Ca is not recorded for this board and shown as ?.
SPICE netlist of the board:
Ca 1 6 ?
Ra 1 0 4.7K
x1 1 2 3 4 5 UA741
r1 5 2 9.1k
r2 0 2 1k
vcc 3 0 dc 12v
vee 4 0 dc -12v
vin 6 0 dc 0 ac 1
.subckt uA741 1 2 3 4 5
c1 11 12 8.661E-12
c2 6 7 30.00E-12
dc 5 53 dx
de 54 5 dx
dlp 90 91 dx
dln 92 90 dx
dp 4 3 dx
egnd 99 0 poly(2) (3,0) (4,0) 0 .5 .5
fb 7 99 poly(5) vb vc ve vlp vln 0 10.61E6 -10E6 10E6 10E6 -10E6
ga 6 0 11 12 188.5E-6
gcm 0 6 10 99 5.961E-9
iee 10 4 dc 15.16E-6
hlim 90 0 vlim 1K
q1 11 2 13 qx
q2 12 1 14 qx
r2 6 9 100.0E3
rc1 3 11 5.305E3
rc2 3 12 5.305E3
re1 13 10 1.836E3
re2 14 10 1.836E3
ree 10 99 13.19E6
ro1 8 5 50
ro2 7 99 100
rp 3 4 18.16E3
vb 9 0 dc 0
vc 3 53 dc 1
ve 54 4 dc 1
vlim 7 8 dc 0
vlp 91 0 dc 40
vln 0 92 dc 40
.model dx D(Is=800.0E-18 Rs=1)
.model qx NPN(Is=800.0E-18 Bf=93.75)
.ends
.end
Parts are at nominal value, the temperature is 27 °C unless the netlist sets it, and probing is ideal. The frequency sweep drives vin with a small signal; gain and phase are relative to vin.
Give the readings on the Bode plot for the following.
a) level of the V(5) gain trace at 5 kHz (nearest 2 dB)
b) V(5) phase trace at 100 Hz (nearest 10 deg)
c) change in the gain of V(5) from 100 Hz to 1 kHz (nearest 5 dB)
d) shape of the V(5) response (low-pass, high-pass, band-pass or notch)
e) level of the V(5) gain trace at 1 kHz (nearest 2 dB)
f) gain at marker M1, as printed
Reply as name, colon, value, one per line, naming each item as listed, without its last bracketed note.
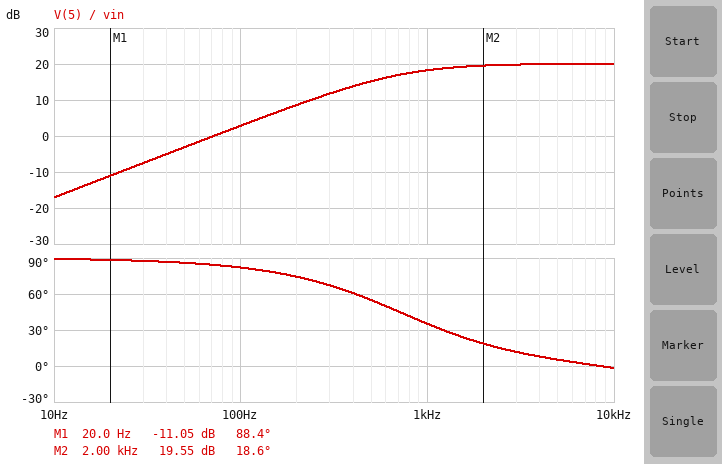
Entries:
level of the V(5) gain trace at 5 kHz: 20 dB
V(5) phase trace at 100 Hz: 80 deg
change in the gain of V(5) from 100 Hz to 1 kHz: 15 dB
shape of the V(5) response: high-pass
level of the V(5) gain trace at 1 kHz: 18 dB
gain at marker M1, as printed: -11.05 dB
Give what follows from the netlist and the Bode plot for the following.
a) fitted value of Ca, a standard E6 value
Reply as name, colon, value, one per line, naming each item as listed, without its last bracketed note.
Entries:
fitted value of Ca, a standard E6 value: 47 nF
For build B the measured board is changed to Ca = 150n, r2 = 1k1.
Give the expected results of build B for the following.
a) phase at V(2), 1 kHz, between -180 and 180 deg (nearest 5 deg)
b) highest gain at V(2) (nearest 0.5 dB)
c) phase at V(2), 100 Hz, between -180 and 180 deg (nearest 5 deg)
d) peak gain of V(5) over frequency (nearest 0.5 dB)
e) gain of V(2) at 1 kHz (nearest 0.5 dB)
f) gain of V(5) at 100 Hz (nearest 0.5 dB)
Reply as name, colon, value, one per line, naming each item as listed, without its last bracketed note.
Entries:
phase at V(2), 1 kHz, between -180 and 180 deg: 10 deg
highest gain at V(2): 0 dB
phase at V(2), 100 Hz, between -180 and 180 deg: 65 deg
peak gain of V(5) over frequency: 19.5 dB
gain of V(2) at 1 kHz: 0 dB
gain of V(5) at 100 Hz: 11.5 dB
